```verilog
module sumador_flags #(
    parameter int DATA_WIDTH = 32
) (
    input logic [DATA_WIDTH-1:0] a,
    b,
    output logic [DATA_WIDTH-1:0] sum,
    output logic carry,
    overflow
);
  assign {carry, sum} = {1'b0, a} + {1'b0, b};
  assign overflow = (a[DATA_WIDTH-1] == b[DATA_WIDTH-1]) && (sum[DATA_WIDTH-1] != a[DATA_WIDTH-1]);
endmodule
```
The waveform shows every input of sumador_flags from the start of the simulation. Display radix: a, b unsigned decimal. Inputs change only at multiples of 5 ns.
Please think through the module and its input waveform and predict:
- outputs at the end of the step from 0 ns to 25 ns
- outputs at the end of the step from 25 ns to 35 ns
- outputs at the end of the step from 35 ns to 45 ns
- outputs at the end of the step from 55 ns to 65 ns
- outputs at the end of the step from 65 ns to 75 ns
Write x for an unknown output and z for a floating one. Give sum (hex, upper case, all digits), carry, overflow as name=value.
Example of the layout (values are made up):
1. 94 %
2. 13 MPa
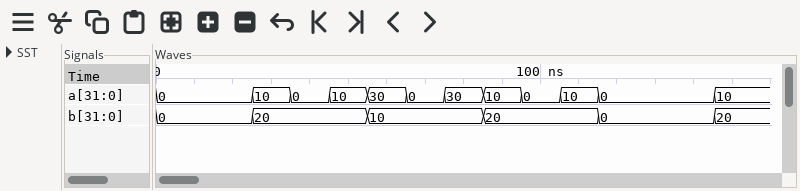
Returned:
1. sum=00000000, carry=0, overflow=0
2. sum=0000001E, carry=0, overflow=0
3. sum=00000014, carry=0, overflow=0
4. sum=00000028, carry=0, overflow=0
5. sum=0000000A, carry=0, overflow=0
